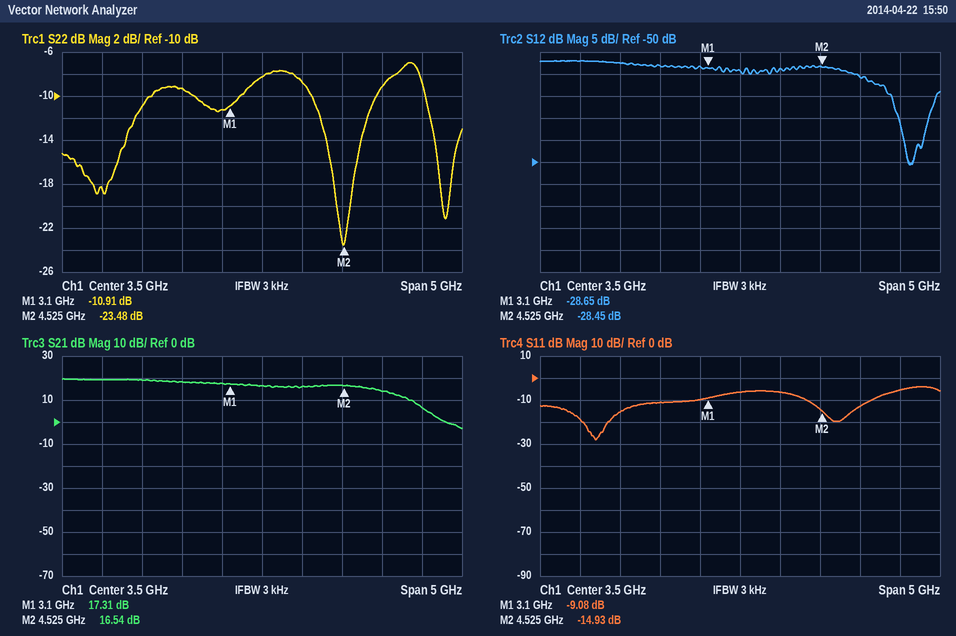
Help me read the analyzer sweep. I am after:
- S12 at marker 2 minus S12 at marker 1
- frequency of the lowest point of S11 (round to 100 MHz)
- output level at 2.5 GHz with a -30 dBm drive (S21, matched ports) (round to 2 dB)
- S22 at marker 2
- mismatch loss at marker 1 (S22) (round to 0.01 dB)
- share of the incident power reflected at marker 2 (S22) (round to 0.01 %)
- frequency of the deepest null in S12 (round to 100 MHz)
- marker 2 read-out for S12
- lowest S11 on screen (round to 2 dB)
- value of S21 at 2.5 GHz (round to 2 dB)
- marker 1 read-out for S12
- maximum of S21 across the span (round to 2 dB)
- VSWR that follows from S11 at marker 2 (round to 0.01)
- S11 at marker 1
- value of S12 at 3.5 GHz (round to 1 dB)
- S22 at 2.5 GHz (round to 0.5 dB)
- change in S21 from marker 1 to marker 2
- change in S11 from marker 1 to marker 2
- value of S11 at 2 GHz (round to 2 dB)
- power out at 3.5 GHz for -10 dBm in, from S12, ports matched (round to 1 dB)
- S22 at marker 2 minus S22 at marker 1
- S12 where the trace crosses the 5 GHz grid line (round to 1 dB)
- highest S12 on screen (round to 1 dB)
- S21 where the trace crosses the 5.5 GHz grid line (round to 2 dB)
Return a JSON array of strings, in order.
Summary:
["0.20 dB", "1.7 GHz", "-12 dBm", "-23.48 dB", "0.37 dB", "0.45 %", "5.6 GHz", "-28.45 dB", "-28 dB", "18 dB", "-28.65 dB", "20 dB", "1.44", "-9.08 dB", "-29 dB", "-9.5 dB", "-0.77 dB", "-5.85 dB", "-16 dB", "-39 dBm", "-12.57 dB", "-31 dB", "-27 dB", "6 dB"]
